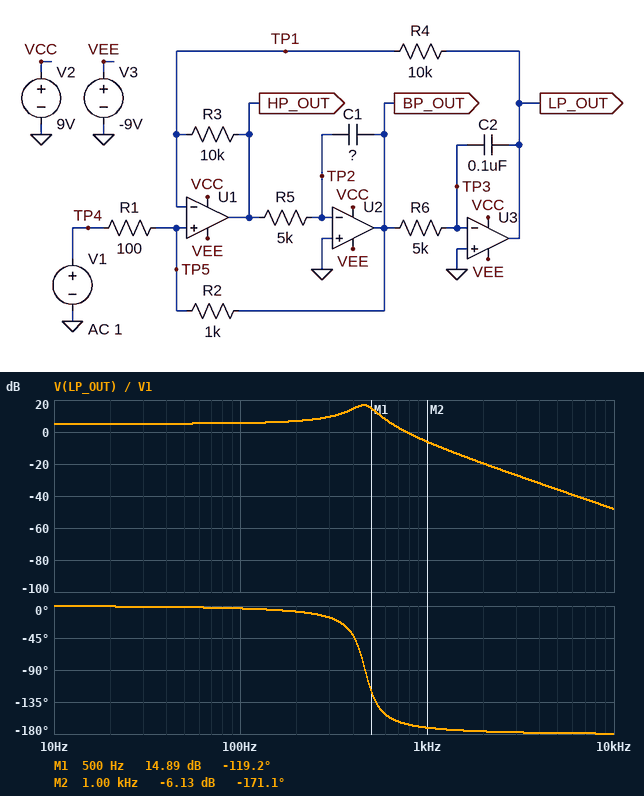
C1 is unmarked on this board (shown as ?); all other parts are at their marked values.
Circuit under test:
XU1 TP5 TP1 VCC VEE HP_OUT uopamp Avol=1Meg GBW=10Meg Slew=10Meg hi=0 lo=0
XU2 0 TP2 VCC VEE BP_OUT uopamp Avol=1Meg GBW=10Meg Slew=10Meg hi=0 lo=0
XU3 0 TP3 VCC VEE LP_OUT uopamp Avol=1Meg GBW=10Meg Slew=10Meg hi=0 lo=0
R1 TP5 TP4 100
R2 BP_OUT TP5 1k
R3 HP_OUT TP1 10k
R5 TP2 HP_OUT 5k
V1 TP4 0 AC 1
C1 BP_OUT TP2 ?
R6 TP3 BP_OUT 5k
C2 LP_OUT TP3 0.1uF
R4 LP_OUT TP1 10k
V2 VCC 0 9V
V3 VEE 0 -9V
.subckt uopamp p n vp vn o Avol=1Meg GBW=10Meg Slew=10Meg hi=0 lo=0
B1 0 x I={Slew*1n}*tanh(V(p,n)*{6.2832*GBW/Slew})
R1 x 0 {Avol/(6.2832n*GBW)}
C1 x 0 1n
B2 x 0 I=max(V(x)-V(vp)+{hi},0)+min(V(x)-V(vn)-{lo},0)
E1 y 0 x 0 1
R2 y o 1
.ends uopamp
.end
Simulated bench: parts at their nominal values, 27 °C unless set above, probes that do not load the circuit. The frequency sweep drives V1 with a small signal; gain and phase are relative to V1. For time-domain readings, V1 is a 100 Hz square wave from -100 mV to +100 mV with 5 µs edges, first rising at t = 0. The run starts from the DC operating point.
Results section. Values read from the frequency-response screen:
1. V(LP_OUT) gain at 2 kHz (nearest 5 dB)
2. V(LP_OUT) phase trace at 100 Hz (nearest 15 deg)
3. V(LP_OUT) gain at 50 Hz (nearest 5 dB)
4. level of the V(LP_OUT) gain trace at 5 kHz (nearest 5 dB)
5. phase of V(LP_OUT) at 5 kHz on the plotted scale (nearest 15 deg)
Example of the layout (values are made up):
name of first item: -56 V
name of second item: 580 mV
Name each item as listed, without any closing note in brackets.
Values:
V(LP_OUT) gain at 2 kHz: -20 dB
V(LP_OUT) phase trace at 100 Hz: 0 deg
V(LP_OUT) gain at 50 Hz: 5 dB
level of the V(LP_OUT) gain trace at 5 kHz: -35 dB
phase of V(LP_OUT) at 5 kHz on the plotted scale: -180 deg
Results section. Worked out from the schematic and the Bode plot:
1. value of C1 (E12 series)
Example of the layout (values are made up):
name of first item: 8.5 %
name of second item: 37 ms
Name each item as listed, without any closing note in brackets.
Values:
value of C1: 47 nF
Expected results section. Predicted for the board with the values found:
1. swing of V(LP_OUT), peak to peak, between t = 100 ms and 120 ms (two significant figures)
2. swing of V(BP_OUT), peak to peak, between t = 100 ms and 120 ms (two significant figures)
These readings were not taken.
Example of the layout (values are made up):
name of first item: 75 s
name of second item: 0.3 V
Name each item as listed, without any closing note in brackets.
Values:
swing of V(LP_OUT), peak to peak, between t = 100 ms and 120 ms: 850 mV
swing of V(BP_OUT), peak to peak, between t = 100 ms and 120 ms: 890 mV
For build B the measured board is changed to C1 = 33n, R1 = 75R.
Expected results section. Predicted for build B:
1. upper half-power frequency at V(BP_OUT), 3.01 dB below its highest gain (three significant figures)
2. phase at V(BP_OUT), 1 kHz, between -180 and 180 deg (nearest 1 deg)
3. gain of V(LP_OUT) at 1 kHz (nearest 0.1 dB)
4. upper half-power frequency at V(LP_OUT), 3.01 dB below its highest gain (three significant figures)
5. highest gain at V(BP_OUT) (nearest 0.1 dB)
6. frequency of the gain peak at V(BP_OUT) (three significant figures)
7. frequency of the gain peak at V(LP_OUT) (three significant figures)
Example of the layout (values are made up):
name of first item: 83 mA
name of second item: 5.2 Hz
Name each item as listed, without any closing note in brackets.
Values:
upper half-power frequency at V(BP_OUT), 3.01 dB below its highest gain: 625 Hz
phase at V(BP_OUT), 1 kHz, between -180 and 180 deg: 101 deg
gain of V(LP_OUT) at 1 kHz: -1.8 dB
upper half-power frequency at V(LP_OUT), 3.01 dB below its highest gain: 610 Hz
highest gain at V(BP_OUT): 22.5 dB
frequency of the gain peak at V(BP_OUT): 554 Hz
frequency of the gain peak at V(LP_OUT): 546 Hz
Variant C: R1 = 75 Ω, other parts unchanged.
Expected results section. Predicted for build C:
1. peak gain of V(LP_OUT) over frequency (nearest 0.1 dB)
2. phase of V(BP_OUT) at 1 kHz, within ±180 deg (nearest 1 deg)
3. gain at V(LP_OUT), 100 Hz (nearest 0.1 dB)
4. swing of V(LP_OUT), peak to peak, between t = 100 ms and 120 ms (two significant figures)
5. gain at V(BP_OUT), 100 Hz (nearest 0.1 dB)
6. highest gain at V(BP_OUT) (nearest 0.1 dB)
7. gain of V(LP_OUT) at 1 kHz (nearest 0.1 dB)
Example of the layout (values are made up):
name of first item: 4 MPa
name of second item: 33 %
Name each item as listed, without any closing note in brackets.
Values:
peak gain of V(LP_OUT) over frequency: 19.3 dB
phase of V(BP_OUT) at 1 kHz, within ±180 deg: 97 deg
gain at V(LP_OUT), 100 Hz: 5.8 dB
swing of V(LP_OUT), peak to peak, between t = 100 ms and 120 ms: 930 mV
gain at V(BP_OUT), 100 Hz: -4.3 dB
highest gain at V(BP_OUT): 22.5 dB
gain of V(LP_OUT) at 1 kHz: -5.9 dB
